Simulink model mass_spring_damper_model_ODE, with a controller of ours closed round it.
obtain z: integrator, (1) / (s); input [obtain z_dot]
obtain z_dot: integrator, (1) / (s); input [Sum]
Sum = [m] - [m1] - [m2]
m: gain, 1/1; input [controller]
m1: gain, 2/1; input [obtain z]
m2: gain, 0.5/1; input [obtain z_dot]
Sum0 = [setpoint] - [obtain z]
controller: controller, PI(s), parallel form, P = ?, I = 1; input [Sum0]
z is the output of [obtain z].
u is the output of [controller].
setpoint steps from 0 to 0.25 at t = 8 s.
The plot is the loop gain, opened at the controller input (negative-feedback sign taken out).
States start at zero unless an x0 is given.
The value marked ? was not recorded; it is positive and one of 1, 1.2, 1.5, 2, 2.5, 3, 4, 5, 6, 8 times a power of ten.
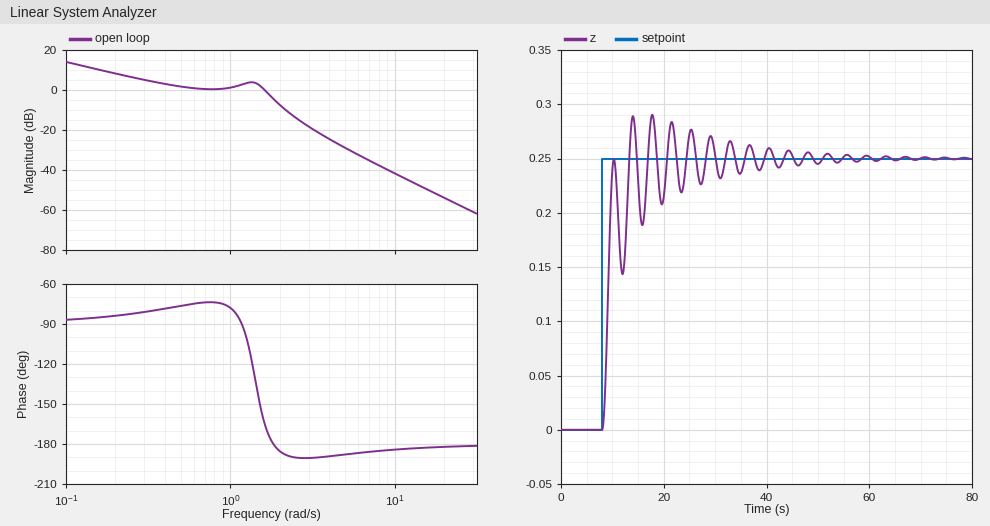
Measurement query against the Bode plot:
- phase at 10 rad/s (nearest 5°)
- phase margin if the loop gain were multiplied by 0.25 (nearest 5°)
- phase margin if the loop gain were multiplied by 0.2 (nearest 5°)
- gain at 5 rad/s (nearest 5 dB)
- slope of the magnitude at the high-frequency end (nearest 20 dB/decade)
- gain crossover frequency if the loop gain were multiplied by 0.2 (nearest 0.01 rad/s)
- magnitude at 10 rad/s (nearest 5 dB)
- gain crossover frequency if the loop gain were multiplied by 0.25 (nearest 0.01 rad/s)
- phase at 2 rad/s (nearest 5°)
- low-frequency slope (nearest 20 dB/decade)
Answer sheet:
-185°
95°
95°
-30 dB
-40 dB/decade
0.10 rad/s
-40 dB
0.13 rad/s
-185°
-20 dB/decade
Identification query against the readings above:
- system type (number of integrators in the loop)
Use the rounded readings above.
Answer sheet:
1
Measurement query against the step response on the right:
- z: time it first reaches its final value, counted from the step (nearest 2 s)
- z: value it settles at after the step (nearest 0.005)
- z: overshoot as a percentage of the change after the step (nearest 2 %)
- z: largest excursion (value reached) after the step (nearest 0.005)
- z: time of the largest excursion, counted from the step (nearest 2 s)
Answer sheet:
6 s
0.250
16 %
0.290
10 s
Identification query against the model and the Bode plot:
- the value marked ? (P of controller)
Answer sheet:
0.8
